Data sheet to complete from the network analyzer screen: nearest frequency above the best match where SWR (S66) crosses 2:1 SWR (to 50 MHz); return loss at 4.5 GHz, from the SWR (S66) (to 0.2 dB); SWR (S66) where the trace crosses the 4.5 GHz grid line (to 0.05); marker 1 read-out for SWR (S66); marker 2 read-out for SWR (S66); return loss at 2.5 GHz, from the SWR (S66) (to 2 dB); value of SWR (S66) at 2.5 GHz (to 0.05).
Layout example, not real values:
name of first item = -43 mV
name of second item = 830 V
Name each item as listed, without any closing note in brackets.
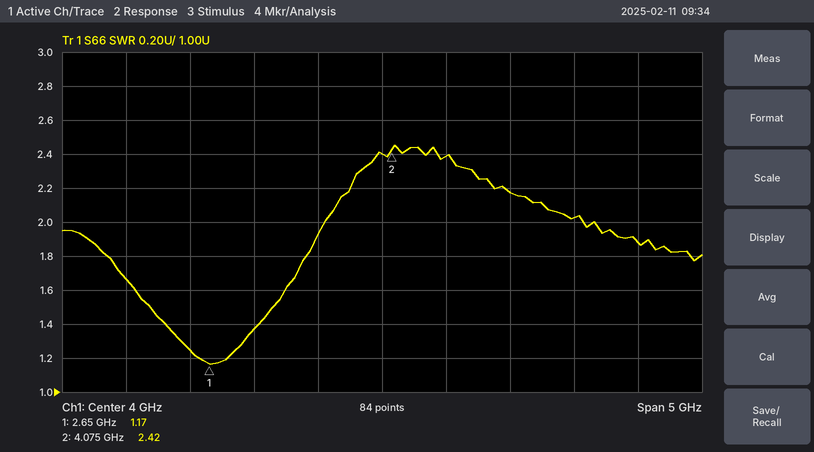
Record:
nearest frequency above the best match where SWR (S66) crosses 2:1 SWR = 3.55 GHz
return loss at 4.5 GHz, from the SWR (S66) = 7.8 dB
SWR (S66) where the trace crosses the 4.5 GHz grid line = 2.40
marker 1 read-out for SWR = 1.17
marker 2 read-out for SWR = 2.42
return loss at 2.5 GHz, from the SWR (S66) = 20 dB
value of SWR (S66) at 2.5 GHz = 1.25
